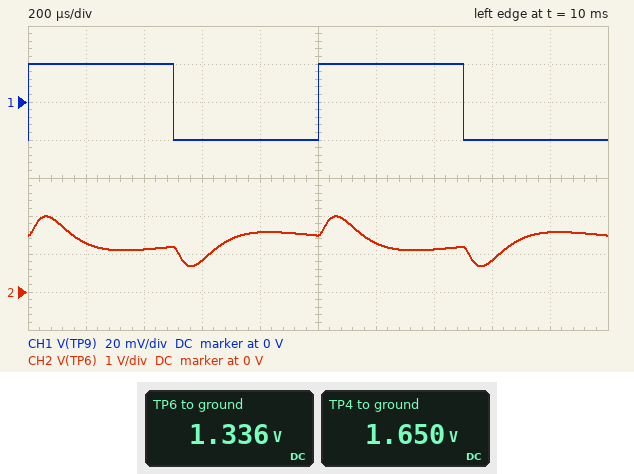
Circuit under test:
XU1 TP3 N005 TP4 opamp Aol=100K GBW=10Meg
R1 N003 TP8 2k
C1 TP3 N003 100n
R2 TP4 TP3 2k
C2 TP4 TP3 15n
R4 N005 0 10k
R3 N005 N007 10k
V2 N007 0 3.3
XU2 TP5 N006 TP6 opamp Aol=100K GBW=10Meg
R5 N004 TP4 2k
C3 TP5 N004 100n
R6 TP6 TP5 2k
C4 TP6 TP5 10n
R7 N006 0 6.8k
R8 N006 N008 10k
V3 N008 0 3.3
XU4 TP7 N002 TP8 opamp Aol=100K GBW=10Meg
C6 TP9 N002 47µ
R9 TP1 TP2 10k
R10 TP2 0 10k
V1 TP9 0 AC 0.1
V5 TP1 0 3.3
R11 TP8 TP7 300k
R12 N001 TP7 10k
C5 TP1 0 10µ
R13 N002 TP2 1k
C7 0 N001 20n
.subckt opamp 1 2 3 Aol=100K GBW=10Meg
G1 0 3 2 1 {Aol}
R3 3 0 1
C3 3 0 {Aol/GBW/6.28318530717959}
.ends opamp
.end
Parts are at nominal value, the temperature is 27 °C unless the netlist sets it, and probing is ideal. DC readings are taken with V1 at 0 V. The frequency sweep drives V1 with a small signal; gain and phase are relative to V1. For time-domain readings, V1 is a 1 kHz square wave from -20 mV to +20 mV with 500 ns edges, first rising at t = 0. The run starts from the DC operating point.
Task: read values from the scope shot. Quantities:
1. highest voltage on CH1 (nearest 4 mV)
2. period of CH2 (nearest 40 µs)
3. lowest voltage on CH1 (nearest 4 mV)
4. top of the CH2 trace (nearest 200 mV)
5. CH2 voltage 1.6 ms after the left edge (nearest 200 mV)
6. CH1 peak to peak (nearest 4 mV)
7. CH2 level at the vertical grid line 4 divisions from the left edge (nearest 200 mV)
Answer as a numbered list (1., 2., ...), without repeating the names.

1. 20 mV
2. 1.00 ms
3. -20 mV
4. 2.0 V
5. 800 mV
6. 40 mV
7. 1.6 V
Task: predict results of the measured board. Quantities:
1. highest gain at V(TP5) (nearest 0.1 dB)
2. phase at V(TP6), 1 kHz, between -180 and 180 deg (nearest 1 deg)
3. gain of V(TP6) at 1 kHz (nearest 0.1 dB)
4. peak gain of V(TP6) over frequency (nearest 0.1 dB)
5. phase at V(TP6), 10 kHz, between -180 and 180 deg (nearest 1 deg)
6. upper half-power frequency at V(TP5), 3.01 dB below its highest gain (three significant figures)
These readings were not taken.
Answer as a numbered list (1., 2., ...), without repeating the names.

1. -40.3 dB
2. 96 deg
3. 23.2 dB
4. 27.3 dB
5. -102 deg
6. 16.3 kHz
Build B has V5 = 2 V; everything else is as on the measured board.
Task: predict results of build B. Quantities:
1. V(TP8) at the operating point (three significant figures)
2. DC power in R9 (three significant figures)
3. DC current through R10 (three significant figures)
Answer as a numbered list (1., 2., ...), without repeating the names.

1. 1.00 V
2. 100 µW
3. 100 µA
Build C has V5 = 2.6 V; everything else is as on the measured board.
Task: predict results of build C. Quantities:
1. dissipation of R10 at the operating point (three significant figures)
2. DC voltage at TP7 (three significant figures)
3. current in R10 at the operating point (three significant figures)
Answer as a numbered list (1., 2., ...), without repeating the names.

1. 169 µW
2. 1.30 V
3. 130 µA
